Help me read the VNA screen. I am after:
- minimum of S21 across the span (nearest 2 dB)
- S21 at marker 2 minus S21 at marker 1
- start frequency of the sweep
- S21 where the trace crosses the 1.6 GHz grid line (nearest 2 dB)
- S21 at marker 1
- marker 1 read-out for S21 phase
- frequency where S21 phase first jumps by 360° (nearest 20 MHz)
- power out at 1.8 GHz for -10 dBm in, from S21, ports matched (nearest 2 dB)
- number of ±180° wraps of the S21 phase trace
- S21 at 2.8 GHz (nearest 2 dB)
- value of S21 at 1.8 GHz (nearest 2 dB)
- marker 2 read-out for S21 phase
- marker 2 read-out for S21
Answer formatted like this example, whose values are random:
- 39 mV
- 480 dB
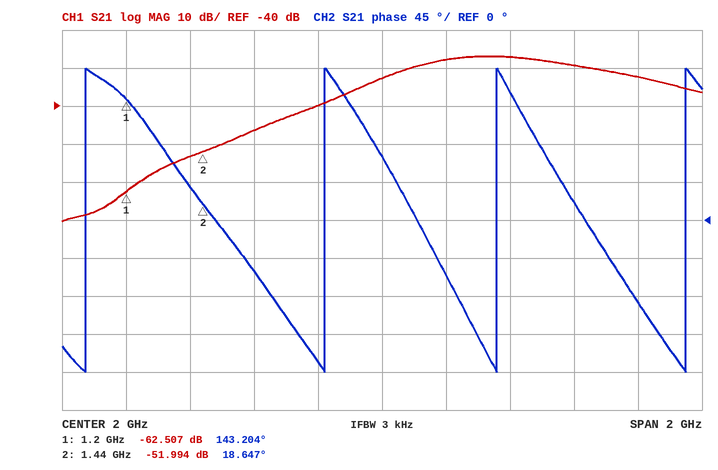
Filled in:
- -70 dB
- 10.513 dB
- 1 GHz
- -46 dB
- -62.507 dB
- 143.204°
- 1.08 GHz
- -50 dBm
- 4
- -32 dB
- -40 dB
- 18.647°
- -51.994 dB
